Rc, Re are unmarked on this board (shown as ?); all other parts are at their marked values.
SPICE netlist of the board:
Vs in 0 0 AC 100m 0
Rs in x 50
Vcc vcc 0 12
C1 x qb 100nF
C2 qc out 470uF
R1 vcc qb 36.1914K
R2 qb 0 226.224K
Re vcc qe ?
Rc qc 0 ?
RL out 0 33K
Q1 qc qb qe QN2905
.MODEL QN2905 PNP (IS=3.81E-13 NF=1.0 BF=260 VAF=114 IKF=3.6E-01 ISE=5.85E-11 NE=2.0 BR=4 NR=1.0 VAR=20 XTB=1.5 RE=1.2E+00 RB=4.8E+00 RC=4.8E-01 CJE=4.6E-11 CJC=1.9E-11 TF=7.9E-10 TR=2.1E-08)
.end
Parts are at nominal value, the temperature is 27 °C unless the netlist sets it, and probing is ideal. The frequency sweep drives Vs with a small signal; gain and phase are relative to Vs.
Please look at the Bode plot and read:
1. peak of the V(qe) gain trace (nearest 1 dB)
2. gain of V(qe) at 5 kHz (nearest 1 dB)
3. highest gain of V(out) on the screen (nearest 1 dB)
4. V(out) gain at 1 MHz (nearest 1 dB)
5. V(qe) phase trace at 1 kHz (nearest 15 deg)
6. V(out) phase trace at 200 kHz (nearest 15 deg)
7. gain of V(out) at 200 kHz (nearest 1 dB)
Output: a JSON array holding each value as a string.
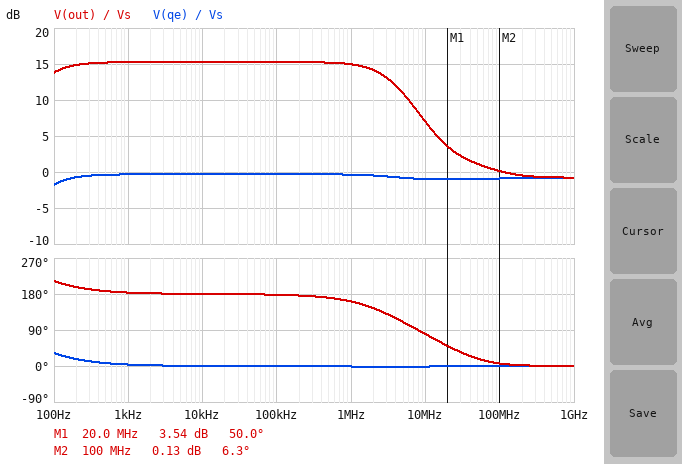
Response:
["0 dB", "0 dB", "15 dB", "15 dB", "0 deg", "180 deg", "15 dB"]
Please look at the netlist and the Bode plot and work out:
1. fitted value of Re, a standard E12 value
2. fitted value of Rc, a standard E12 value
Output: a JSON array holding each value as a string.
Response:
["680 Ω", "4.7 kΩ"]
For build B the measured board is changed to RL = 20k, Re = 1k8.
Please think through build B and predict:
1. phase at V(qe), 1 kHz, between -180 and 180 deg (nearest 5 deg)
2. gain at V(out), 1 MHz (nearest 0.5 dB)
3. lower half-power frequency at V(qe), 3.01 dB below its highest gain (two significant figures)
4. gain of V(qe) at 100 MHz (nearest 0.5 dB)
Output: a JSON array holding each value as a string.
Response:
["5 deg", "6.0 dB", "56 Hz", "-0.5 dB"]
